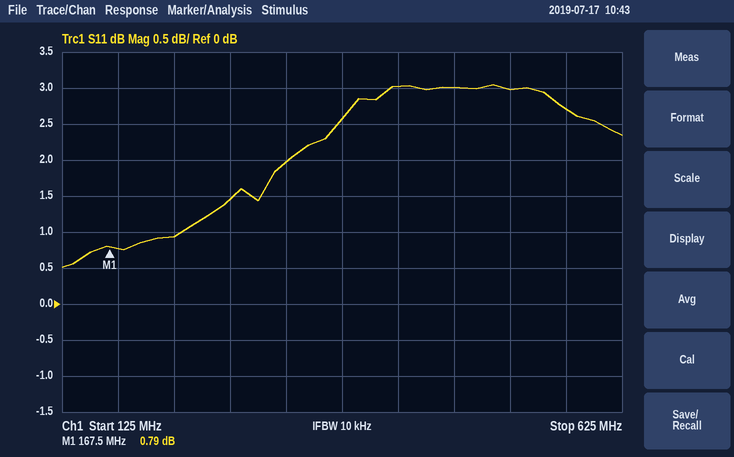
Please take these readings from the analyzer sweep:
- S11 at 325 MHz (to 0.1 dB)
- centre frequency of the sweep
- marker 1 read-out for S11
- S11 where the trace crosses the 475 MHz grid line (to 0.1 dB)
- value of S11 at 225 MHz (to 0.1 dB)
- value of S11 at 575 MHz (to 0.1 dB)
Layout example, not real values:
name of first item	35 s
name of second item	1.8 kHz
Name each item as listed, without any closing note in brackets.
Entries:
S11 at 325 MHz	2.0 dB
centre frequency of the sweep	375 MHz
marker 1 read-out for S11	0.79 dB
S11 where the trace crosses the 475 MHz grid line	3.0 dB
value of S11 at 225 MHz	0.9 dB
value of S11 at 575 MHz	2.7 dB
